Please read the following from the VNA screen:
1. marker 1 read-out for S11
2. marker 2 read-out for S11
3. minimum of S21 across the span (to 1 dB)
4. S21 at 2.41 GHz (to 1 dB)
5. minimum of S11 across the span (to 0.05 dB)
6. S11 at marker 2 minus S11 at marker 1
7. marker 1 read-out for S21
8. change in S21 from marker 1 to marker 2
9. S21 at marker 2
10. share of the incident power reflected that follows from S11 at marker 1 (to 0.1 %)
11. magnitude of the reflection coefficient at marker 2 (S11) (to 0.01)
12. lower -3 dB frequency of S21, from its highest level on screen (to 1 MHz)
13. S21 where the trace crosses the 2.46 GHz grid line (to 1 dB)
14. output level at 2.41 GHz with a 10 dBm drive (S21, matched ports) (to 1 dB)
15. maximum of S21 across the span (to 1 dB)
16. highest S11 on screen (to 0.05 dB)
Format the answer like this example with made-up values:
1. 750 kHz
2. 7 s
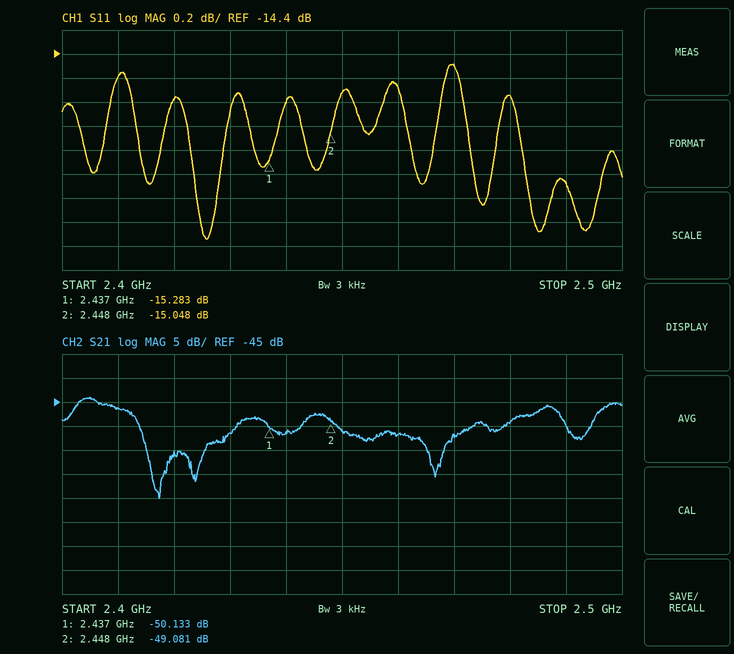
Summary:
1. -15.283 dB
2. -15.048 dB
3. -65 dB
4. -46 dB
5. -15.95 dB
6. 0.235 dB
7. -50.133 dB
8. 1.052 dB
9. -49.081 dB
10. 3.0 %
11. 0.18
12. 2.402 GHz
13. -52 dB
14. -36 dBm
15. -44 dB
16. -14.50 dB
